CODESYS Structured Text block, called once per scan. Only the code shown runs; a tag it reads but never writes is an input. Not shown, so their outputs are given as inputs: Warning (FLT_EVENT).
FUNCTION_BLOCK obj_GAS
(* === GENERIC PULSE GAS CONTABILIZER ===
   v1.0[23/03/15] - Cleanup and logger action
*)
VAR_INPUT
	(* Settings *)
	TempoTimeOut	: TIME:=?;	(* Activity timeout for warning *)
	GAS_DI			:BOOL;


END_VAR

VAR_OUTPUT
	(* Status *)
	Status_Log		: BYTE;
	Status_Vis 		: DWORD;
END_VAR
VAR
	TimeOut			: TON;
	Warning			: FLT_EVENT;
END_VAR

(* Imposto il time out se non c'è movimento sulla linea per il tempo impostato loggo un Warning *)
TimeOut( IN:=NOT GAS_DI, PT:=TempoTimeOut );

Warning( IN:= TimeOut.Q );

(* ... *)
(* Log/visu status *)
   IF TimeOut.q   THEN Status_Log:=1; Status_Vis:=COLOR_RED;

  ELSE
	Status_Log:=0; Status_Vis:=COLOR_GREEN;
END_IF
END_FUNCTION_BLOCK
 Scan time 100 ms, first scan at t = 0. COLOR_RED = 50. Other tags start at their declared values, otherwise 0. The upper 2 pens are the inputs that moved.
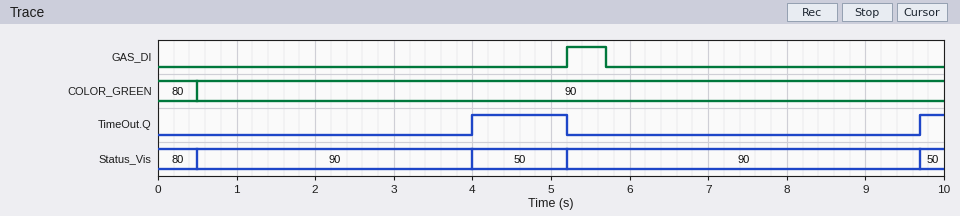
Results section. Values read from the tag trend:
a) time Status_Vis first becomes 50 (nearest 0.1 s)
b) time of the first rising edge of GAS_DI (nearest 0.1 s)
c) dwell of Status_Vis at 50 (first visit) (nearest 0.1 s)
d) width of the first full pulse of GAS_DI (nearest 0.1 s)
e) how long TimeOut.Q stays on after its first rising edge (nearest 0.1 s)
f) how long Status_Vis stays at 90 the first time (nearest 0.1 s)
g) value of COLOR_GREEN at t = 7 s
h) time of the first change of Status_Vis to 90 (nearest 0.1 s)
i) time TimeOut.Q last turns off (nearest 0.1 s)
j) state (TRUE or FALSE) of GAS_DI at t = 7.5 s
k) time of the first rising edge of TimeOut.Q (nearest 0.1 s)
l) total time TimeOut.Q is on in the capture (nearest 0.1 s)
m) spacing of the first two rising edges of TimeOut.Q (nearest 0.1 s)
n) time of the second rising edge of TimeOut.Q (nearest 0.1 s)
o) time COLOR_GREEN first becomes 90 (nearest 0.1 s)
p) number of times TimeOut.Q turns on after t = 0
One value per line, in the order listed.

4.0 s
5.2 s
1.2 s
0.5 s
1.2 s
3.5 s
90
0.5 s
5.2 s
FALSE
4.0 s
1.5 s
5.7 s
9.7 s
0.5 s
2
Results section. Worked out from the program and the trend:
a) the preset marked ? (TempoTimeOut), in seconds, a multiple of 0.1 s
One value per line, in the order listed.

4.0 s
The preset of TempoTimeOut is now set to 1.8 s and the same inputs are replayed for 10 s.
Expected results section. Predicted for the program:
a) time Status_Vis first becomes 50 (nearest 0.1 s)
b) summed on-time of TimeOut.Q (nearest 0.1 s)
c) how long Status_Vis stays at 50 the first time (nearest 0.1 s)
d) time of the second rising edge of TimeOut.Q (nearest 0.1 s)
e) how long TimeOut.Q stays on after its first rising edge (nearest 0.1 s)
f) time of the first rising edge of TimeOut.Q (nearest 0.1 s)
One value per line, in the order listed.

1.8 s
5.9 s
3.4 s
7.5 s
3.4 s
1.8 s
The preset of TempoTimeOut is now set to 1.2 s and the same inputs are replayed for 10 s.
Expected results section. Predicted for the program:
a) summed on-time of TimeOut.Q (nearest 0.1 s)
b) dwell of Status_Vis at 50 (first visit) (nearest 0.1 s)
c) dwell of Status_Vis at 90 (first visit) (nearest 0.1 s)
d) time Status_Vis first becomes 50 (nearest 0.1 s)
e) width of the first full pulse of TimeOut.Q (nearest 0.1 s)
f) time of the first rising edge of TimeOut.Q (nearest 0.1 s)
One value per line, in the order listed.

7.1 s
4.0 s
0.7 s
1.2 s
4.0 s
1.2 s
